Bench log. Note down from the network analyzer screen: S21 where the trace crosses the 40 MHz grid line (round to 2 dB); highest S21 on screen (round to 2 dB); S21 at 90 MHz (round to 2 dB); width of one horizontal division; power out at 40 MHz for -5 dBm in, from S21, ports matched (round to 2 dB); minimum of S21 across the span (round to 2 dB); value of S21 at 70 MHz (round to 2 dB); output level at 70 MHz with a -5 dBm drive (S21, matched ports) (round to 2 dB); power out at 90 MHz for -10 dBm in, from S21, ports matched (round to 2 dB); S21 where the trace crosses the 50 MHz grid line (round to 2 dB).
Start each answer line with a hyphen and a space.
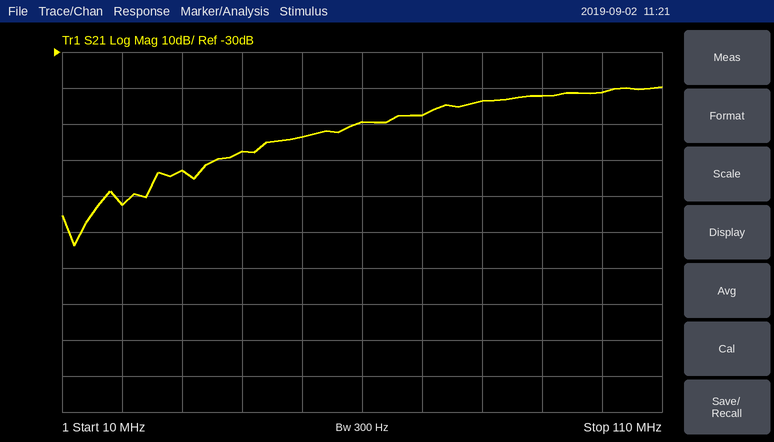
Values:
- -58 dB
- -40 dB
- -42 dB
- 10 MHz
- -62 dBm
- -84 dB
- -48 dB
- -52 dBm
- -52 dBm
- -54 dB
